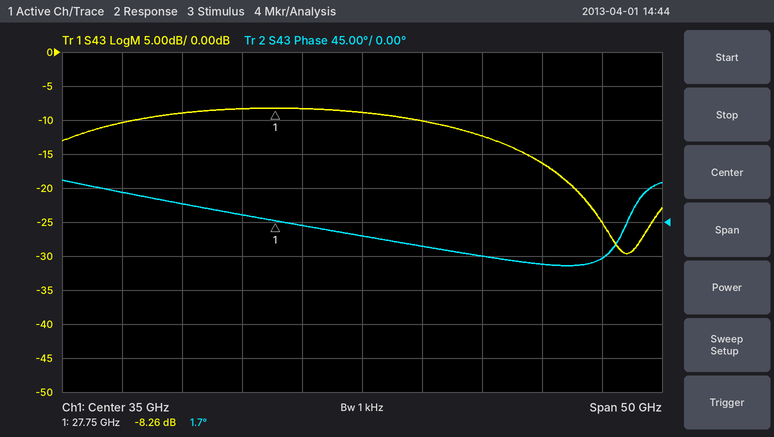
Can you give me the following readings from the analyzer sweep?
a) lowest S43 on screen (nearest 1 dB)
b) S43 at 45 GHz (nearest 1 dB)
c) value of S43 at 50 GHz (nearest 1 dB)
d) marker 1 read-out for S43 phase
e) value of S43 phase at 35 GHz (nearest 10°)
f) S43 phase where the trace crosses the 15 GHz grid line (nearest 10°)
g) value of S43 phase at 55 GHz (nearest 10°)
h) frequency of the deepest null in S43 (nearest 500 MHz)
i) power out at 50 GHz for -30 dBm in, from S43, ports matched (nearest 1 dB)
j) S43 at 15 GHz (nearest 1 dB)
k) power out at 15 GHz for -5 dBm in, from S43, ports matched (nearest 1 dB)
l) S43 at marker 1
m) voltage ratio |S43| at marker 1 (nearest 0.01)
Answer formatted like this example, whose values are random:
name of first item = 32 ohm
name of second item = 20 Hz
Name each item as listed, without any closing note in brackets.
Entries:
lowest S43 on screen = -30 dB
S43 at 45 GHz = -12 dB
value of S43 at 50 GHz = -16 dB
marker 1 read-out for S43 phase = 1.7°
value of S43 phase at 35 GHz = -20°
S43 phase where the trace crosses the 15 GHz grid line = 40°
value of S43 phase at 55 GHz = -50°
frequency of the deepest null in S43 = 57.0 GHz
power out at 50 GHz for -30 dBm in, from S43, ports matched = -46 dBm
S43 at 15 GHz = -10 dB
power out at 15 GHz for -5 dBm in, from S43, ports matched = -15 dBm
S43 at marker 1 = -8.26 dB
voltage ratio |S43| at marker 1 = 0.39
